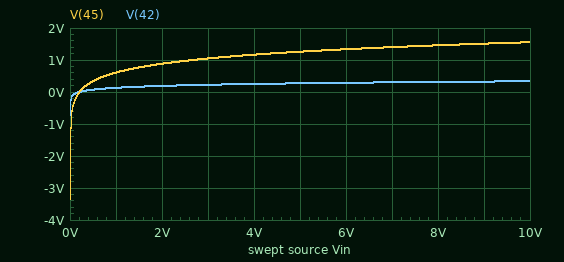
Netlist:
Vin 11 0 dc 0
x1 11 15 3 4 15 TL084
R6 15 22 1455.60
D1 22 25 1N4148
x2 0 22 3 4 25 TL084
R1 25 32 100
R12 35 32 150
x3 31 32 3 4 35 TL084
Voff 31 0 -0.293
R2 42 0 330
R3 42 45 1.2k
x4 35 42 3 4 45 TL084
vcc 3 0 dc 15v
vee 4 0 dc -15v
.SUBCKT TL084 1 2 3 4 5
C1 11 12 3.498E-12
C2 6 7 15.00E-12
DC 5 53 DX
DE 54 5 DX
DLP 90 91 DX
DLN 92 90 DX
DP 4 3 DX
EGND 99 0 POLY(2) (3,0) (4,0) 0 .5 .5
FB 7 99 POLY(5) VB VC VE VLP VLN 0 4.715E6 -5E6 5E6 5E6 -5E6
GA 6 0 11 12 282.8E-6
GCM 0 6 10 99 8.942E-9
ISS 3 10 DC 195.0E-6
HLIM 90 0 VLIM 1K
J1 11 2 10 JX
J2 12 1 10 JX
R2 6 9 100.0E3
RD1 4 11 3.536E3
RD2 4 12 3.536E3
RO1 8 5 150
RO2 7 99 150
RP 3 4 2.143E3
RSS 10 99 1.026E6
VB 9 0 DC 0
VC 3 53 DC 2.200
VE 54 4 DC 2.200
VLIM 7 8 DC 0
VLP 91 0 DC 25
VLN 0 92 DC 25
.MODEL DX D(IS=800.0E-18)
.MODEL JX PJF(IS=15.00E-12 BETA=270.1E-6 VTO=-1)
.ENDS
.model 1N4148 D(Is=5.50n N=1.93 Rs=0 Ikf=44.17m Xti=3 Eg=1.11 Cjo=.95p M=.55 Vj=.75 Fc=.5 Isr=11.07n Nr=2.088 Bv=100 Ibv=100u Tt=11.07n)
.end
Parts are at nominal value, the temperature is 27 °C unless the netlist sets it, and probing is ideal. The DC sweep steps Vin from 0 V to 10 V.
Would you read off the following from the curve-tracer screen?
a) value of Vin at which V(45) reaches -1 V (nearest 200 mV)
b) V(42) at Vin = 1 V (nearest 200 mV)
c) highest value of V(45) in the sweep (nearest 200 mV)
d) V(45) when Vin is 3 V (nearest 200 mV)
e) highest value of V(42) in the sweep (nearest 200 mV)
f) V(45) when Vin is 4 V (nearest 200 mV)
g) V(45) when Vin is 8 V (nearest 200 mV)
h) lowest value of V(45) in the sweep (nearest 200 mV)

0 V
200 mV
1.6 V
1.0 V
400 mV
1.2 V
1.4 V
-3.4 V
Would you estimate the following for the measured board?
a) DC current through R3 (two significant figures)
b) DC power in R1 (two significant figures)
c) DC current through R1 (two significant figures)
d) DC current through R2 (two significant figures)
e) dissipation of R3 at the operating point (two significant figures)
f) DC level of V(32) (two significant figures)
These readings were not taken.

2.2 mA
820 µW
2.9 mA
2.2 mA
5.7 mW
-290 mV
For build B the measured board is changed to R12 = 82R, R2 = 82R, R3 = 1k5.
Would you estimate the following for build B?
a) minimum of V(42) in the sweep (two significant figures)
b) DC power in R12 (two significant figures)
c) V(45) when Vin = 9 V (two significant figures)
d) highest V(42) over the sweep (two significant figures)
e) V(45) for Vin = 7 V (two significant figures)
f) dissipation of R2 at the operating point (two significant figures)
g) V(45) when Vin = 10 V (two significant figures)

-530 mV
670 µW
870 mV
51 mV
630 mV
3.4 mW
980 mV
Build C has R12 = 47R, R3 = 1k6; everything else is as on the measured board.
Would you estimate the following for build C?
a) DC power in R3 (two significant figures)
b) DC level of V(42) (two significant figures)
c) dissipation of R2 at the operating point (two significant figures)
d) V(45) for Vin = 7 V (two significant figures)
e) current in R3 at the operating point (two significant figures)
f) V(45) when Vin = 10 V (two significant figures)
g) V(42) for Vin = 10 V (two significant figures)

2.7 mW
-430 mV
550 µW
-620 mV
1.3 mA
-560 mV
-96 mV
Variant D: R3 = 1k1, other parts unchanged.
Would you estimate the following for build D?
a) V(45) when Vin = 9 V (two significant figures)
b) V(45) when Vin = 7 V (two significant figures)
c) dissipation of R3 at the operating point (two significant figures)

1.4 V
1.3 V
5.3 mW
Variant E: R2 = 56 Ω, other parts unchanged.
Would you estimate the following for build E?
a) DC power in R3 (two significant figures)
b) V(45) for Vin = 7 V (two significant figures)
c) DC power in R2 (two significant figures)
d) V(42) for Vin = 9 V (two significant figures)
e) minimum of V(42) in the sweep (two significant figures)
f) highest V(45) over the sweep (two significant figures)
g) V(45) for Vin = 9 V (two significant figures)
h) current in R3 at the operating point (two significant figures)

140 mW
6.8 V
6.4 mW
330 mV
-600 mV
7.5 V
7.3 V
11 mA
